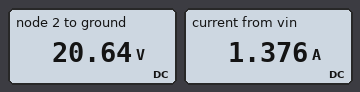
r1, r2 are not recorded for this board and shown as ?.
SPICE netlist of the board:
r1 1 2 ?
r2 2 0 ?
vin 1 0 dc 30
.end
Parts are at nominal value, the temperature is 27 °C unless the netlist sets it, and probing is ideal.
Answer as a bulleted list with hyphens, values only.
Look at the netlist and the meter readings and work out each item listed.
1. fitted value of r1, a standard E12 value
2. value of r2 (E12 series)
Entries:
- 6.8 Ω
- 15 Ω
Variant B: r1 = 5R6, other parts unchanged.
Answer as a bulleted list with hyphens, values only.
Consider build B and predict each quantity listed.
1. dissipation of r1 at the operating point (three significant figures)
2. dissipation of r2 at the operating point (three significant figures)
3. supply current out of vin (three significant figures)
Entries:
- 11.9 W
- 31.8 W
- 1.46 A
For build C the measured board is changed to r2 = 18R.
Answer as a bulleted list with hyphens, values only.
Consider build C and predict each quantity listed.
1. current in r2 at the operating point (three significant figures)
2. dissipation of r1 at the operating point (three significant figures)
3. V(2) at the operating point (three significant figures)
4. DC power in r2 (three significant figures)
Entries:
- 1.21 A
- 9.95 W
- 21.8 V
- 26.3 W
